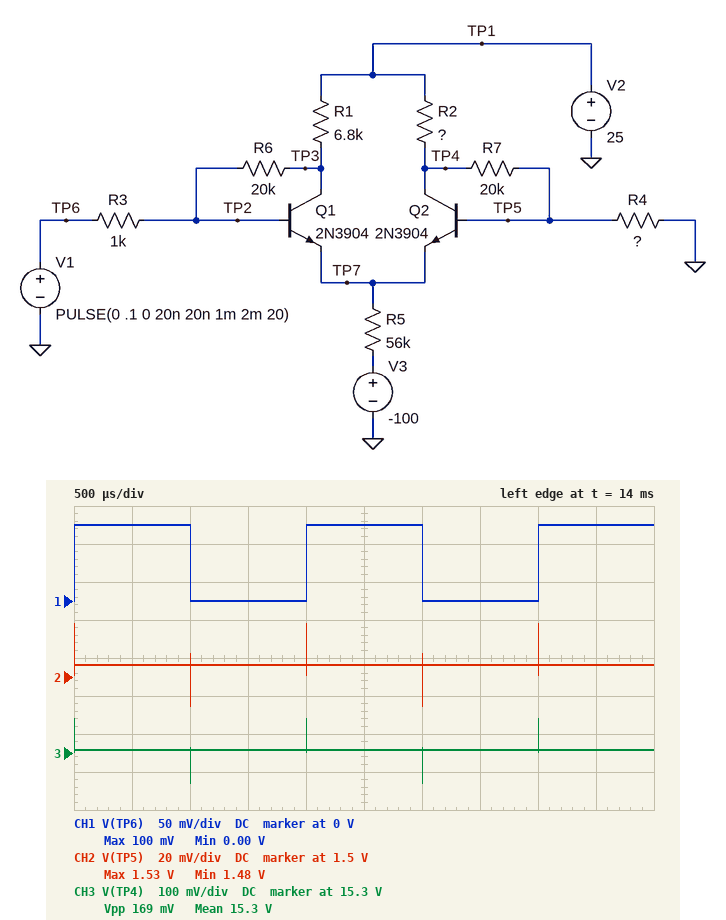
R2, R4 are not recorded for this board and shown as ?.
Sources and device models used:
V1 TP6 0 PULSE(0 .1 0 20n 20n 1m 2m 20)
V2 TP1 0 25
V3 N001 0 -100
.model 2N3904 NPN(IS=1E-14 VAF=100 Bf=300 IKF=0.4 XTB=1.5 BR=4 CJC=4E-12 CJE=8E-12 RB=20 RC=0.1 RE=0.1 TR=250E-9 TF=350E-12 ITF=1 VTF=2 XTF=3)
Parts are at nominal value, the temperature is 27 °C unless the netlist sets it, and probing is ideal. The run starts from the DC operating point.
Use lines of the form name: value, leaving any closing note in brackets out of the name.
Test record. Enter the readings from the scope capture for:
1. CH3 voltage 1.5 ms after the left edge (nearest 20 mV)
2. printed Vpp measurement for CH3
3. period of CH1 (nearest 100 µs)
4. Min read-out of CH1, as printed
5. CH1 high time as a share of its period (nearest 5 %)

CH3 voltage 1.5 ms after the left edge: 15.30 V
printed Vpp measurement for CH3: 169 mV
period of CH1: 2.0 ms
Min read-out of CH1, as printed: 0.00 V
CH1 high time as a share of its period: 50 %
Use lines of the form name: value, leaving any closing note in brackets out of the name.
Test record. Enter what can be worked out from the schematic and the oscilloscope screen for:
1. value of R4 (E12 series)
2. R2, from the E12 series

value of R4: 2.2 kΩ
R2, from the E12 series: 3.9 kΩ
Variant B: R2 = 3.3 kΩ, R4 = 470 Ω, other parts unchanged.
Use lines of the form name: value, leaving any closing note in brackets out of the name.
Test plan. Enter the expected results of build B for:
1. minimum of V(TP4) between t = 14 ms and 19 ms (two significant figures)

minimum of V(TP4) between t = 14 ms and 19 ms: 21 V
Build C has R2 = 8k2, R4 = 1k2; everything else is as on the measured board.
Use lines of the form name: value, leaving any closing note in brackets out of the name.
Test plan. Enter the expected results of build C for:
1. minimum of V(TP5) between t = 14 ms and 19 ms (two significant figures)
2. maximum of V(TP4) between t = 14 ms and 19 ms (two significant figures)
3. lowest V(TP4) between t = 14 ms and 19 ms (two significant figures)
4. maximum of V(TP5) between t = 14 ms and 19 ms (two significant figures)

minimum of V(TP5) between t = 14 ms and 19 ms: 700 mV
maximum of V(TP4) between t = 14 ms and 19 ms: 13 V
lowest V(TP4) between t = 14 ms and 19 ms: 12 V
maximum of V(TP5) between t = 14 ms and 19 ms: 750 mV
